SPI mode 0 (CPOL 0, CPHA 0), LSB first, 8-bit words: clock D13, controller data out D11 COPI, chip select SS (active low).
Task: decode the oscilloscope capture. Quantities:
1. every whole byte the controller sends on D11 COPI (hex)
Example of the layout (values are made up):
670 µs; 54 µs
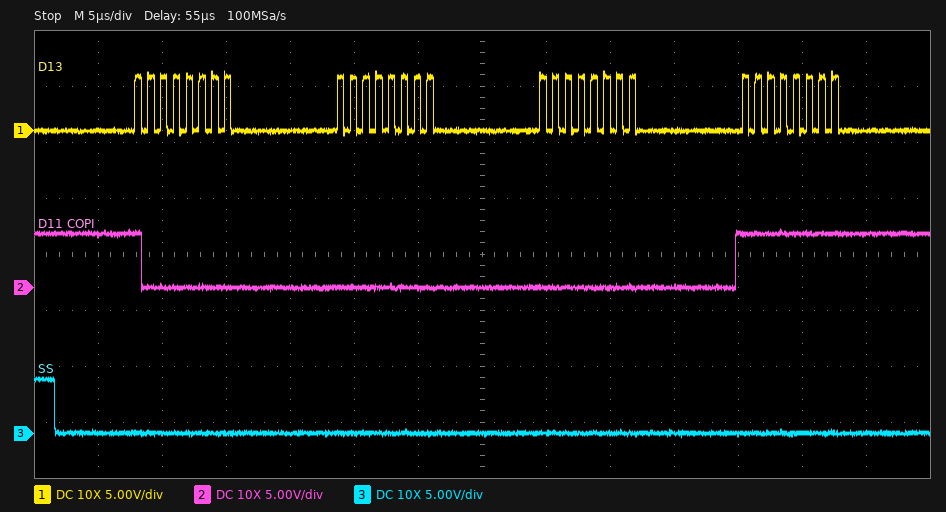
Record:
01 00 00 FF
